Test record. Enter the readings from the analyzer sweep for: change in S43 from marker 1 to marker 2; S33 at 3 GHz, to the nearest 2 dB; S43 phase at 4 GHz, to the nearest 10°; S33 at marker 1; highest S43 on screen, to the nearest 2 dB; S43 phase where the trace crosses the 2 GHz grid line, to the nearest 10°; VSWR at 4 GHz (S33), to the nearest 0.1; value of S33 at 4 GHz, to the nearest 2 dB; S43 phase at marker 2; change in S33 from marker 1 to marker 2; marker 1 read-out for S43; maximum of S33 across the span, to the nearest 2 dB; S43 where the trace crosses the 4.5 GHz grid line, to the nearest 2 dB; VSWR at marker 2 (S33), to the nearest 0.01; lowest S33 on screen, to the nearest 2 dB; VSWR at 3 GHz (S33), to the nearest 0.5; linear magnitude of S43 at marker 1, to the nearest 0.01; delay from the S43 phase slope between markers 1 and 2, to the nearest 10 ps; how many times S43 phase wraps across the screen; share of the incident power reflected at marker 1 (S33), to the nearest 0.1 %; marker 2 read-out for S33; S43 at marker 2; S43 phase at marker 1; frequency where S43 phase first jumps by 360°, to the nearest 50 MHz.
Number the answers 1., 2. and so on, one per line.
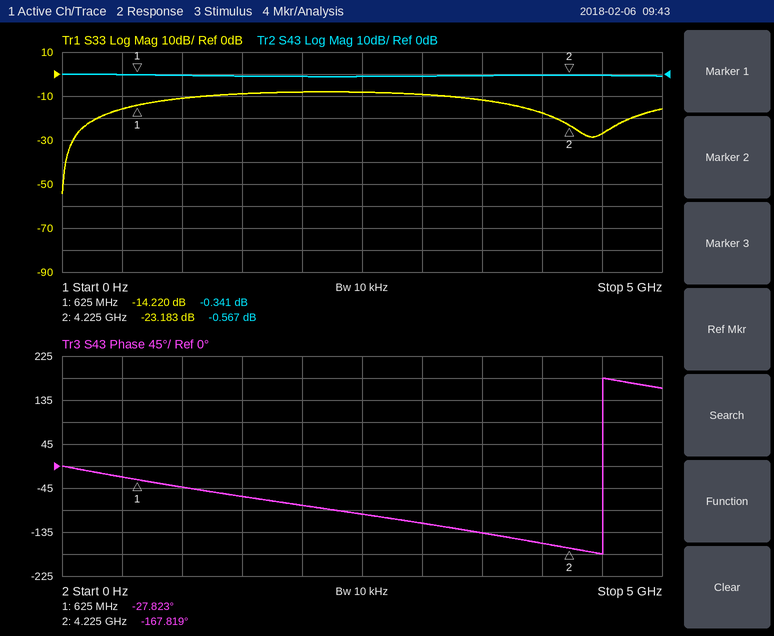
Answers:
1. -0.226 dB
2. -10 dB
3. -160°
4. -14.220 dB
5. 0 dB
6. -80°
7. 1.3
8. -18 dB
9. -167.819°
10. -8.963 dB
11. -0.341 dB
12. -8 dB
13. 0 dB
14. 1.15
15. -54 dB
16. 2.0
17. 0.96
18. 110 ps
19. 1
20. 3.8 %
21. -23.183 dB
22. -0.567 dB
23. -27.823°
24. 4.50 GHz
